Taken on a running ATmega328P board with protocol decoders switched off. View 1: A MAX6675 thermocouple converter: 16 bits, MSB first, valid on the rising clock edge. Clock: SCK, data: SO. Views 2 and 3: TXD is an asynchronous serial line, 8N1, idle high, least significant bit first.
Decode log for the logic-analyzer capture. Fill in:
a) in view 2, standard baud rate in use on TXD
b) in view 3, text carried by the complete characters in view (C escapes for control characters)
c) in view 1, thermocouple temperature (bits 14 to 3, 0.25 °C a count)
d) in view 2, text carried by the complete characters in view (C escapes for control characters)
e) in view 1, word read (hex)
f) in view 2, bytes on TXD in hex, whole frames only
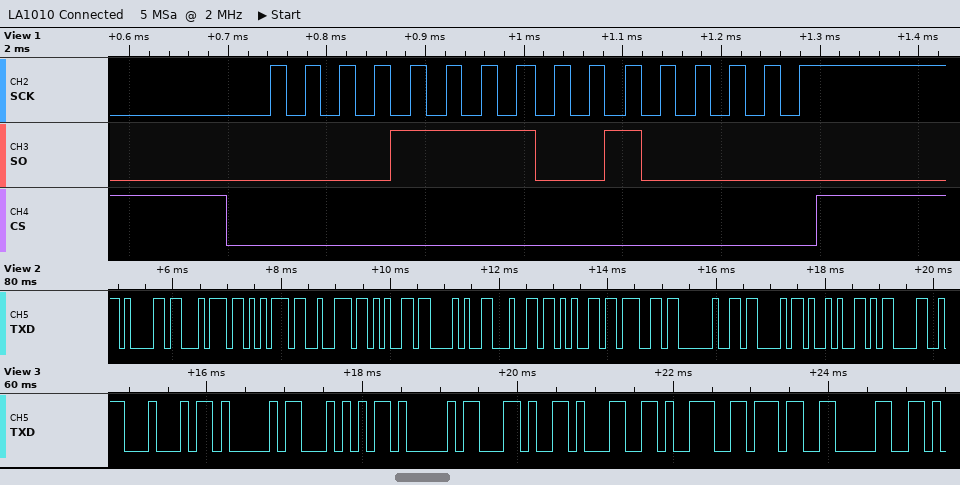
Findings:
9600 baud
"DATA,1970"
121.00 °C
"ature(deg C)\r"
0x0F20
0x61 0x74 0x75 0x72 0x65 0x28 0x64 0x65 0x67 0x20 0x43 0x29 0x0D
